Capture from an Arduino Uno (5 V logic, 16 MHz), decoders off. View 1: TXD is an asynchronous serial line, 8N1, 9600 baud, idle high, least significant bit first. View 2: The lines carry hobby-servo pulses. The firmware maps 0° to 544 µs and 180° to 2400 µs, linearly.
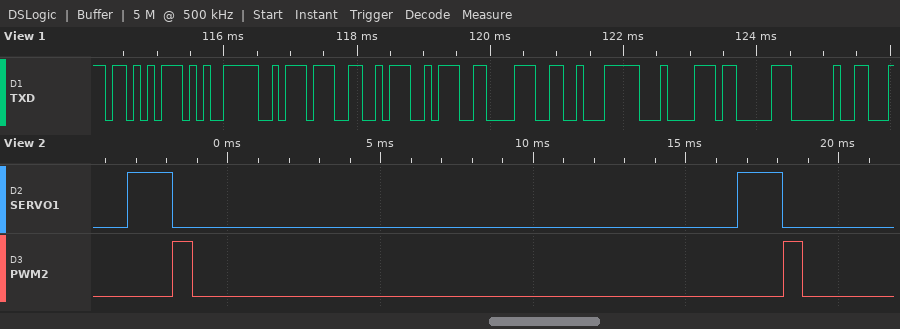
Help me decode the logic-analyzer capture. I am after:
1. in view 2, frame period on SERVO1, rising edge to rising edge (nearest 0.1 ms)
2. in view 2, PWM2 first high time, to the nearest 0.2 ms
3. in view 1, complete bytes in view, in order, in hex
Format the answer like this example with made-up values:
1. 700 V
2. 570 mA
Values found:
1. 20.0 ms
2. 0.6 ms
3. AB E5 BA A6 3A 38 E2 84 83 20
